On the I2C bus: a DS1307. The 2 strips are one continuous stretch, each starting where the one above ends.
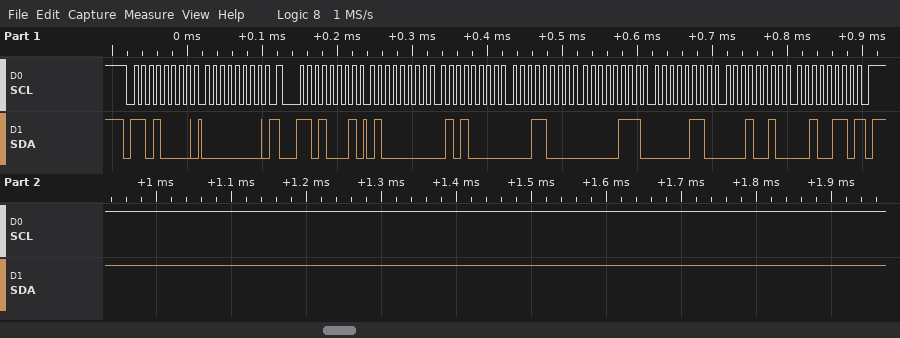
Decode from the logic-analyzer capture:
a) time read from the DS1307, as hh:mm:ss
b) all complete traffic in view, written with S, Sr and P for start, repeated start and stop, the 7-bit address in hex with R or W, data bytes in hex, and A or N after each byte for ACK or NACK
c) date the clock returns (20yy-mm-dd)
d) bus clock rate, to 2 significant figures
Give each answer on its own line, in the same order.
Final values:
18:50:40
S 68W A 00 A Sr 68R A 40 A 50 A 18 A 07 A 06 A 12 A 26 N P
2026-12-06
100 kHz
